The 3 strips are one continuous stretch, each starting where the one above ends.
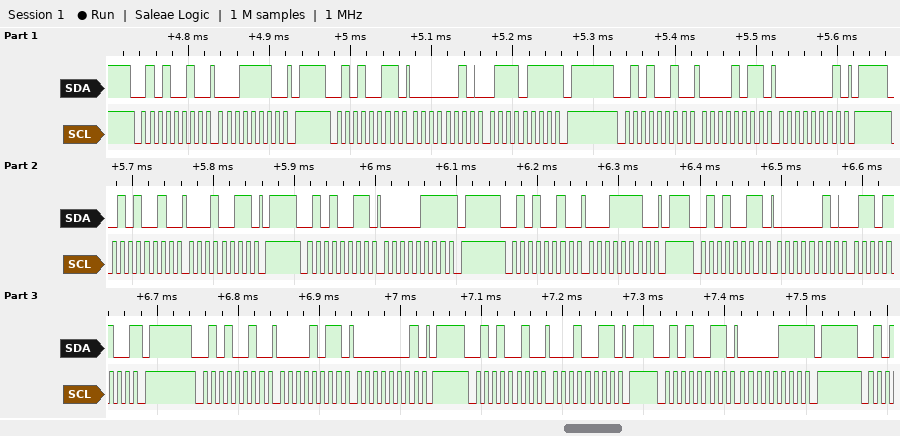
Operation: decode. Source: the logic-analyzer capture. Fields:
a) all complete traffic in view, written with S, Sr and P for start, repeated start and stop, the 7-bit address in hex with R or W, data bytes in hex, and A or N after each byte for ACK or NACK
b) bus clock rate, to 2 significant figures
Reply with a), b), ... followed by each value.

a) S 29W A 1E A P S 29R A 02 A 77 N P S 29W A 0B A 01 A P S 29W A 13 A P S 29R A 07 N P S 29W A 1E A P S 29R A 02 A 6C N P S 29W A 0B A 01 A P S 29W A 13 A P S 29R A 07 N P
b) 100 kHz
